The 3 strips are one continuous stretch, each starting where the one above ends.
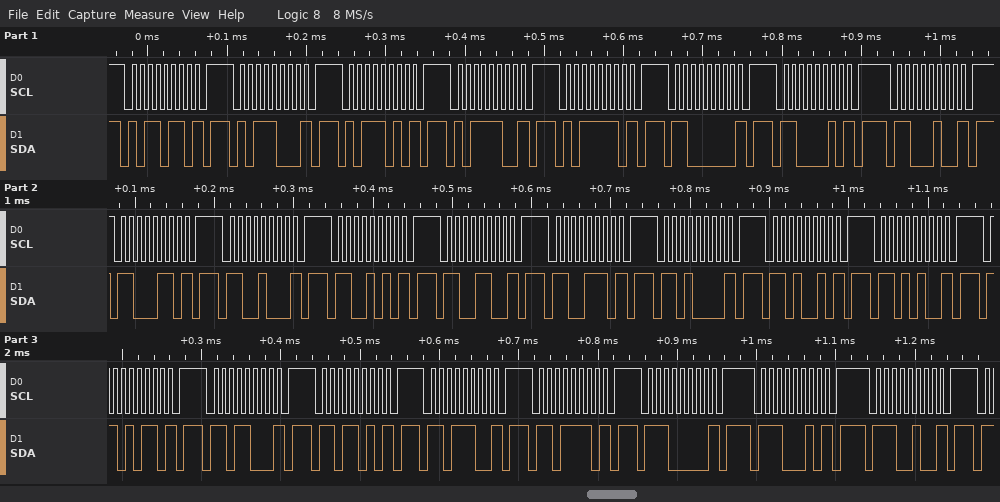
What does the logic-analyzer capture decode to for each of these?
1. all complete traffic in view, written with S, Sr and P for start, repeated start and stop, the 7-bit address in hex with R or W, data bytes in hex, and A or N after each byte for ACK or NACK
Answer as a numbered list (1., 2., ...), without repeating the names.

1. S 5BW N P S 5CW N P S 5DW N P S 5EW N P S 5FW N P S 60W N P S 61W N P S 62W N P S 63W N P S 64W N P S 65W N P S 66W N P S 67W N P S 68W N P S 69W N P S 6AW N P S 6BW N P S 6CW N P S 6DW N P S 6EW N P S 6FW N P S 70W N P S 71W N P S 72W N P
